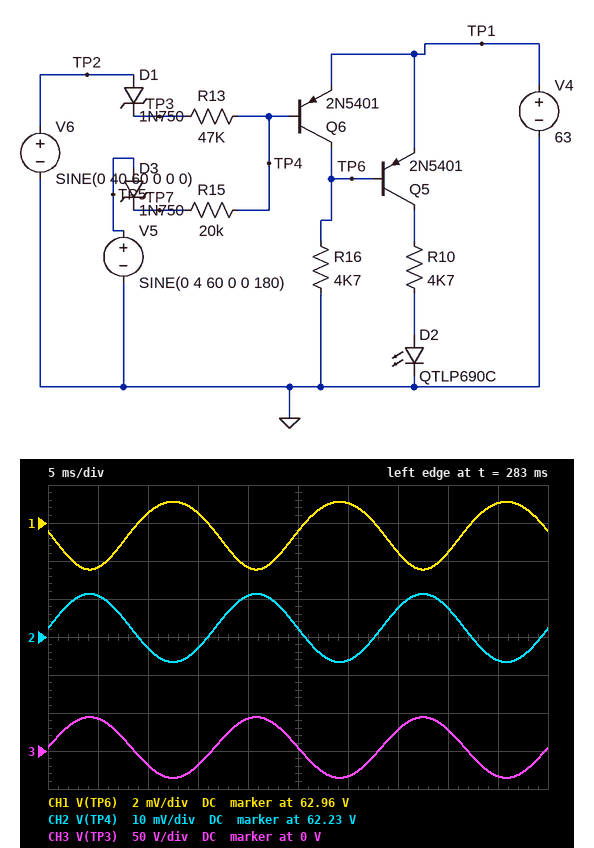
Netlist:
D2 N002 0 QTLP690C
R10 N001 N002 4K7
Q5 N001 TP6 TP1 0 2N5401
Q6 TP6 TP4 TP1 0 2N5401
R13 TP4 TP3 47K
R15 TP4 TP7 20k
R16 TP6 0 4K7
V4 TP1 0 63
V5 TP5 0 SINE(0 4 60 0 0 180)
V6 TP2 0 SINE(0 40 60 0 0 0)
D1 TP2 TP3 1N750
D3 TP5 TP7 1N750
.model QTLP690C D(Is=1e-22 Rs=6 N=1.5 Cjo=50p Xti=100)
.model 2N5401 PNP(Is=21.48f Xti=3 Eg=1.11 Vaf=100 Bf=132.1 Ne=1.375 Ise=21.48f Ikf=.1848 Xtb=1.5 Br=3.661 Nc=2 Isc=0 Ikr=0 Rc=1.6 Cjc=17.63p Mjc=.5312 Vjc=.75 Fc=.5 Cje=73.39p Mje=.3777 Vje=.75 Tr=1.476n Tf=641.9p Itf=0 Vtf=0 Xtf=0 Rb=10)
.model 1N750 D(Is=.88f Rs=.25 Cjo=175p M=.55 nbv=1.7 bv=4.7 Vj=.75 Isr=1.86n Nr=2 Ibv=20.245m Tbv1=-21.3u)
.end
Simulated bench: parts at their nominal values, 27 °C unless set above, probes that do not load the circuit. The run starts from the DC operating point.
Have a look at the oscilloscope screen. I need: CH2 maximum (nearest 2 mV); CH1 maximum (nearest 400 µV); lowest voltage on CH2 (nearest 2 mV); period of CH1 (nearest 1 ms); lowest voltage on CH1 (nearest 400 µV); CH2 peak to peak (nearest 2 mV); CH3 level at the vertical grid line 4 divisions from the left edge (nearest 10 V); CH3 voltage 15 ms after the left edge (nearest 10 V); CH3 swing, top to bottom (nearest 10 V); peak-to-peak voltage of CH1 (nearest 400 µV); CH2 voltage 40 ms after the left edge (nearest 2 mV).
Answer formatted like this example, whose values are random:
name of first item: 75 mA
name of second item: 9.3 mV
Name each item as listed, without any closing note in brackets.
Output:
CH2 maximum: 62.242 V
CH1 maximum: 62.9572 V
lowest voltage on CH2: 62.224 V
period of CH1: 17 ms
lowest voltage on CH1: 62.9536 V
CH2 peak to peak: 18 mV
CH3 level at the vertical grid line 4 divisions from the left edge: 40 V
CH3 voltage 15 ms after the left edge: -20 V
CH3 swing, top to bottom: 80 V
peak-to-peak voltage of CH1: 3.6 mV
CH2 voltage 40 ms after the left edge: 62.238 V
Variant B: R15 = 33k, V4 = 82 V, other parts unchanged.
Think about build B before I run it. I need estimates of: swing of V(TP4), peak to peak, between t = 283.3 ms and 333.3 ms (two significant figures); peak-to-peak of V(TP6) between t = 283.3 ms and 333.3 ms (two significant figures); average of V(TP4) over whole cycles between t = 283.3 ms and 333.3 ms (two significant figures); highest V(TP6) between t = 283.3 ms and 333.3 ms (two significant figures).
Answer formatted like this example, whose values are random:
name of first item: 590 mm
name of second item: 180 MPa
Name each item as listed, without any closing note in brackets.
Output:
swing of V(TP4), peak to peak, between t = 283.3 ms and 333.3 ms: 20 mV
peak-to-peak of V(TP6) between t = 283.3 ms and 333.3 ms: 5.0 mV
average of V(TP4) over whole cycles between t = 283.3 ms and 333.3 ms: 81 V
highest V(TP6) between t = 283.3 ms and 333.3 ms: 82 V
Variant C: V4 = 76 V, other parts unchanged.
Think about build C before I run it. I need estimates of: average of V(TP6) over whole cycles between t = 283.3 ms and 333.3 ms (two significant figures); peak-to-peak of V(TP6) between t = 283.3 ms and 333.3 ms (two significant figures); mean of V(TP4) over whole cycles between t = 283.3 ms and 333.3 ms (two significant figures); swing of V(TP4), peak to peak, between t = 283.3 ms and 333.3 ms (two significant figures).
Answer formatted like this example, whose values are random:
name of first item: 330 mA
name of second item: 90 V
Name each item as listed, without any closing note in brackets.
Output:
average of V(TP6) over whole cycles between t = 283.3 ms and 333.3 ms: 76 V
peak-to-peak of V(TP6) between t = 283.3 ms and 333.3 ms: 2.9 mV
mean of V(TP4) over whole cycles between t = 283.3 ms and 333.3 ms: 75 V
swing of V(TP4), peak to peak, between t = 283.3 ms and 333.3 ms: 17 mV
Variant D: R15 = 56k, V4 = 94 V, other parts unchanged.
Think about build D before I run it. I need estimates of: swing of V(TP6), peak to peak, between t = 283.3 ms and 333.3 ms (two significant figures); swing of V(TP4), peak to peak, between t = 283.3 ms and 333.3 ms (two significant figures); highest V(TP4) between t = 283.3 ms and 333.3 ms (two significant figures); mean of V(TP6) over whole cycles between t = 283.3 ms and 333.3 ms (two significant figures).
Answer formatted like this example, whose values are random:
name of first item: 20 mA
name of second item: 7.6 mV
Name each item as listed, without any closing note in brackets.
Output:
swing of V(TP6), peak to peak, between t = 283.3 ms and 333.3 ms: 7.2 mV
swing of V(TP4), peak to peak, between t = 283.3 ms and 333.3 ms: 21 mV
highest V(TP4) between t = 283.3 ms and 333.3 ms: 93 V
mean of V(TP6) over whole cycles between t = 283.3 ms and 333.3 ms: 94 V
